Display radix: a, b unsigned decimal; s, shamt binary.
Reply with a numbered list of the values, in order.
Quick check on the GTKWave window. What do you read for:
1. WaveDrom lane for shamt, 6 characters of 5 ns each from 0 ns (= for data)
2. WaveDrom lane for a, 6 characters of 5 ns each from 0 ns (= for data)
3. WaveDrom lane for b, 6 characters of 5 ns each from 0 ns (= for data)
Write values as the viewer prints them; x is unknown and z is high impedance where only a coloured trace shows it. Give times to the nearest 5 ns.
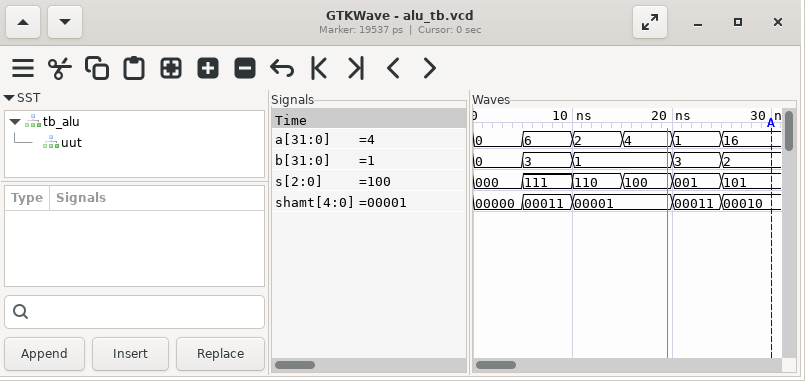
1. {name: 'shamt', wave: '===.==', data: '00000 00011 00001 00011 00010'}
2. {name: 'a', wave: '======', data: '0 6 2 4 1 16'}
3. {name: 'b', wave: '===.==', data: '0 3 1 3 2'}
